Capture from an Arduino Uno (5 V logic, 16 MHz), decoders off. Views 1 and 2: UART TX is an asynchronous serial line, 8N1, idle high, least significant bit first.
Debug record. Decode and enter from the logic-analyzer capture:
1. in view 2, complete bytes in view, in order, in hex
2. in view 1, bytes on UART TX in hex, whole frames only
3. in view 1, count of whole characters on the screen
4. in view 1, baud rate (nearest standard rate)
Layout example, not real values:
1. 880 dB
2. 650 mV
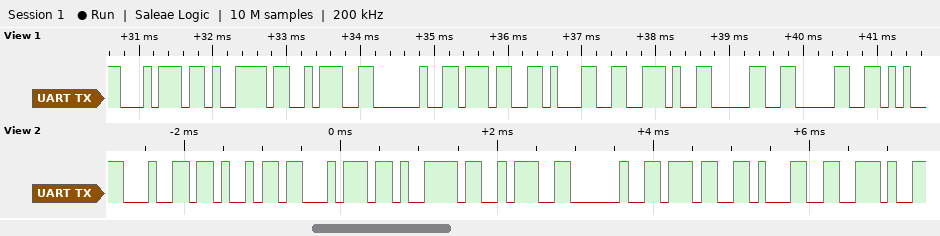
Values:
1. 0x64 0x69 0x74 0x79 0x3A 0x20 0x37 0x31 0x2E
2. 74 79 3A 20 37 31 2E 30 30
3. 9
4. 9600 baud
